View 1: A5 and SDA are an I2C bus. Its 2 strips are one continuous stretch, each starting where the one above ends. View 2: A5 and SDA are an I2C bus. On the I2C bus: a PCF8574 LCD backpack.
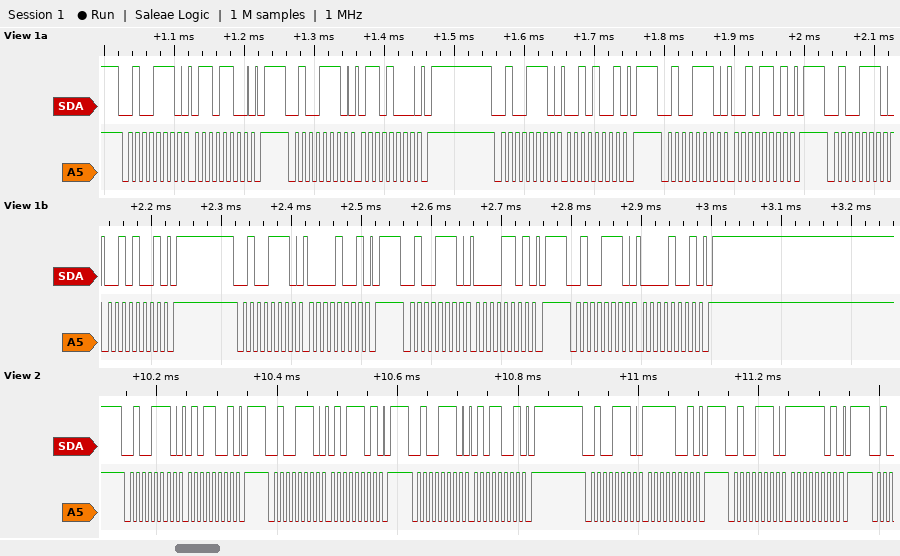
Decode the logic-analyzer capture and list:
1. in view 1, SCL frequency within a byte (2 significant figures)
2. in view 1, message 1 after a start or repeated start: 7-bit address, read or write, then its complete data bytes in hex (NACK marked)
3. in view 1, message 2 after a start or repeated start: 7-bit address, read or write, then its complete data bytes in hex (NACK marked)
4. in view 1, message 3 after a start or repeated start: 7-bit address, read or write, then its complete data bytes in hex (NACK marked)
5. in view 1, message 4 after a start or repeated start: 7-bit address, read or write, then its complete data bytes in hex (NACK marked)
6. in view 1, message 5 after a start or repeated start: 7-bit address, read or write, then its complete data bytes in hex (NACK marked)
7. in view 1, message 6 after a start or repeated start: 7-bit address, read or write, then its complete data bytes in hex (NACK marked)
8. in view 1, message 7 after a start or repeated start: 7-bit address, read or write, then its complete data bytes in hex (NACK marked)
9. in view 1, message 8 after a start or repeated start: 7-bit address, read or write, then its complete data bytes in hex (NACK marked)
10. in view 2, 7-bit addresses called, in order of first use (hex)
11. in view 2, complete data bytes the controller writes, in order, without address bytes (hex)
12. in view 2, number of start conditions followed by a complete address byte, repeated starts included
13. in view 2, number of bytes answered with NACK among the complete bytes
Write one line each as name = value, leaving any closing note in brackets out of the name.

in view 1, SCL frequency within a byte = 100 kHz
in view 1, message 1 after a start or repeated start: 7-bit address, read or write, then its complete data bytes in hex = 0x27 write: 6C
in view 1, message 2 after a start or repeated start: 7-bit address, read or write, then its complete data bytes in hex = 0x27 write: 68
in view 1, message 3 after a start or repeated start: 7-bit address, read or write, then its complete data bytes in hex = 0x27 write: 29
in view 1, message 4 after a start or repeated start: 7-bit address, read or write, then its complete data bytes in hex = 0x27 write: 2D
in view 1, message 5 after a start or repeated start: 7-bit address, read or write, then its complete data bytes in hex = 0x27 write: 29
in view 1, message 6 after a start or repeated start: 7-bit address, read or write, then its complete data bytes in hex = 0x27 write: 09
in view 1, message 7 after a start or repeated start: 7-bit address, read or write, then its complete data bytes in hex = 0x27 write: 0D
in view 1, message 8 after a start or repeated start: 7-bit address, read or write, then its complete data bytes in hex = 0x27 write: 09
in view 2, 7-bit addresses called, in order of first use = 0x27
in view 2, complete data bytes the controller writes, in order, without address bytes = 59 5D 59 F9 FD
in view 2, number of start conditions followed by a complete address byte, repeated starts included = 5
in view 2, number of bytes answered with NACK among the complete bytes = 0
